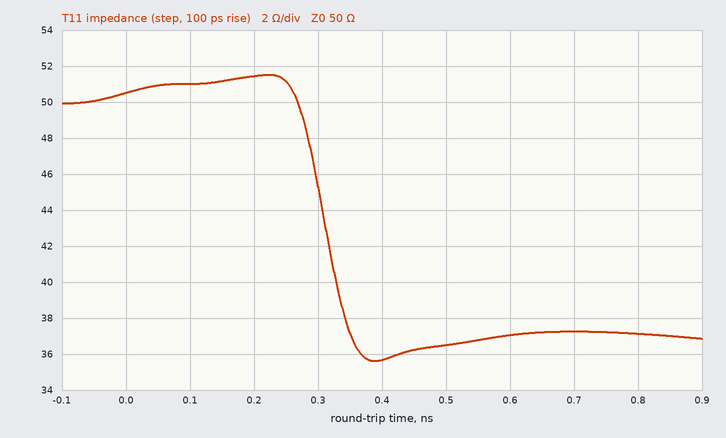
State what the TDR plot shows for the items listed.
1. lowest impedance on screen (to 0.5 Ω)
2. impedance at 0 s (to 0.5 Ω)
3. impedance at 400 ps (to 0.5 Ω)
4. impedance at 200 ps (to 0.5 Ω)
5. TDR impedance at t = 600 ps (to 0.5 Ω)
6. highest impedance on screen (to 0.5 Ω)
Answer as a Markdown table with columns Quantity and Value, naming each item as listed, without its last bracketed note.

| Quantity | Value |
|---|---|
| lowest impedance on screen | 35.5 Ω |
| impedance at 0 s | 50.5 Ω |
| impedance at 400 ps | 35.5 Ω |
| impedance at 200 ps | 51.5 Ω |
| TDR impedance at t = 600 ps | 37.0 Ω |
| highest impedance on screen | 51.5 Ω |
